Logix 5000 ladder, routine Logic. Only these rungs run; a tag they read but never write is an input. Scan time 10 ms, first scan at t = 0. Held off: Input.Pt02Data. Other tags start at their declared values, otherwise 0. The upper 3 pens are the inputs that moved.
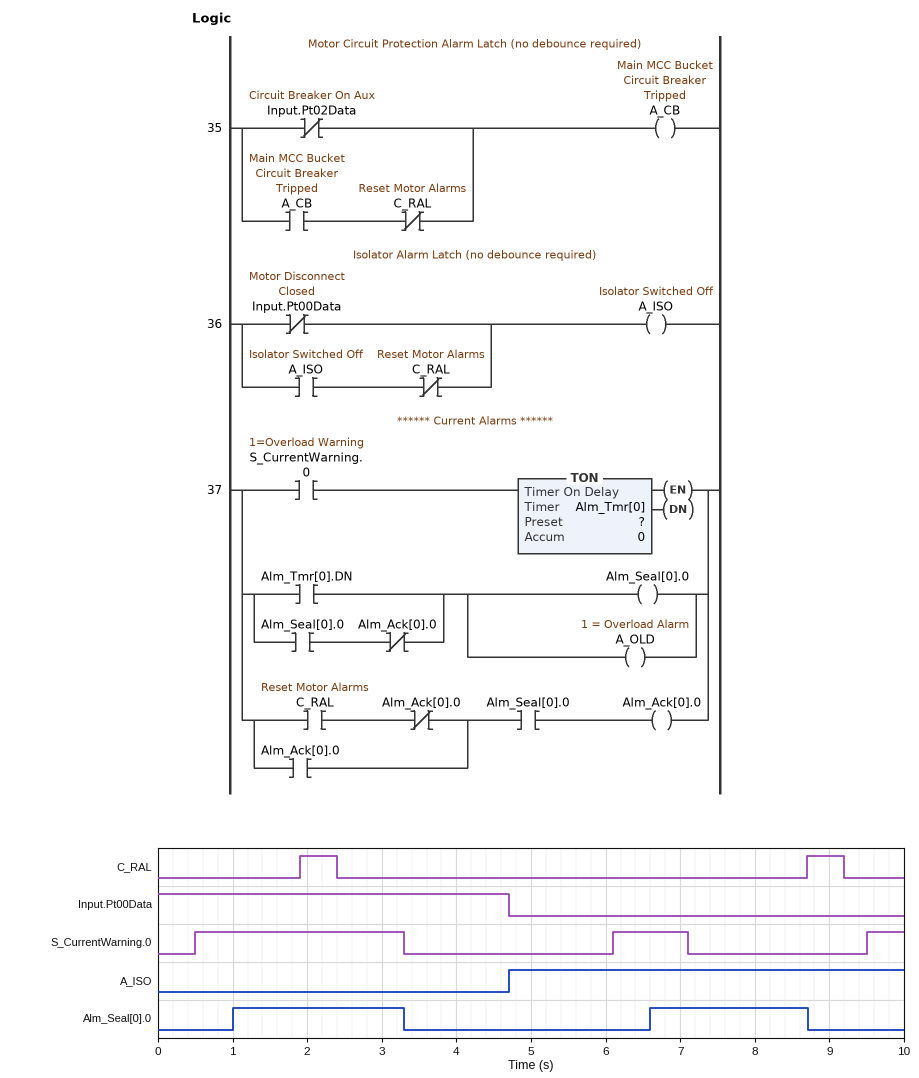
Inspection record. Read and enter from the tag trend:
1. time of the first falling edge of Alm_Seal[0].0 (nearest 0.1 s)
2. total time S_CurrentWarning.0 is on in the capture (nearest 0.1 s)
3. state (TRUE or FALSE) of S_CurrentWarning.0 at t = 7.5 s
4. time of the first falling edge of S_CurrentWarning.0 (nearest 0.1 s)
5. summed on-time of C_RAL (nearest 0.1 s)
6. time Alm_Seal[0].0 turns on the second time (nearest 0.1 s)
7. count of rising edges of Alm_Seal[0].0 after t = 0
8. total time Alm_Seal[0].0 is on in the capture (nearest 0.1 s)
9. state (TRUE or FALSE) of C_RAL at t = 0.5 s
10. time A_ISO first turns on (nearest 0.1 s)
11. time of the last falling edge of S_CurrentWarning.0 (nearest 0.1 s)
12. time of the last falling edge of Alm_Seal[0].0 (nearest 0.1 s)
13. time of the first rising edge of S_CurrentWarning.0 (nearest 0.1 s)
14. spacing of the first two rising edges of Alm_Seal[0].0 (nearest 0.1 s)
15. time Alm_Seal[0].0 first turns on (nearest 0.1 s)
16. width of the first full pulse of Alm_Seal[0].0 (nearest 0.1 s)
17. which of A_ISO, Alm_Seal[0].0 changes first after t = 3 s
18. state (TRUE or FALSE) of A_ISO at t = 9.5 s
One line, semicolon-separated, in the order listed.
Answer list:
3.3 s; 4.3 s; FALSE; 3.3 s; 1.0 s; 6.6 s; 2; 4.4 s; FALSE; 4.7 s; 7.1 s; 8.7 s; 0.5 s; 5.6 s; 1.0 s; 2.3 s; Alm_Seal[0].0; TRUE
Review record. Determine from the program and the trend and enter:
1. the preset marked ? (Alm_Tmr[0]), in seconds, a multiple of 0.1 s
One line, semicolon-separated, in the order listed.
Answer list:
0.5 s
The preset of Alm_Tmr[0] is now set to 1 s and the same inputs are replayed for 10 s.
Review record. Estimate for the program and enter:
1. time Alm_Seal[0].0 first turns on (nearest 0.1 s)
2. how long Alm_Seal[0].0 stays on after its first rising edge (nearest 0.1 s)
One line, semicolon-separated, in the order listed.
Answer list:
1.5 s; 1.8 s
